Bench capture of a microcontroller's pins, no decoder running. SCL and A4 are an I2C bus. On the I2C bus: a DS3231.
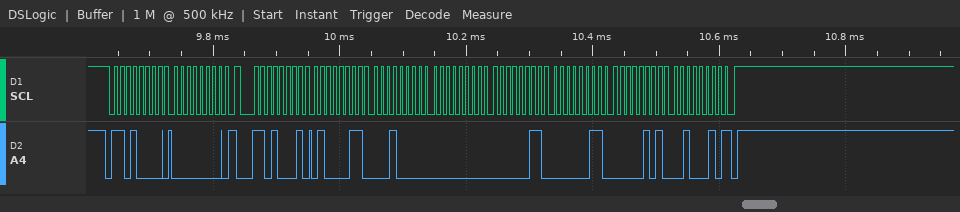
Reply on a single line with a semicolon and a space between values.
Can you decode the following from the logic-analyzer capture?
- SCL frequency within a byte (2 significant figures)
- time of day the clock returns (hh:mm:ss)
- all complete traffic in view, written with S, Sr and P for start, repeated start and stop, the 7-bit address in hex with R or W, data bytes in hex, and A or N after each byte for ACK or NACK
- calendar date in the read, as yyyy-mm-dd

100 kHz; 00:10:43; S 68W A 00 A Sr 68R A 43 A 10 A 00 A 03 A 03 A 05 A 22 N P; 2022-05-03
